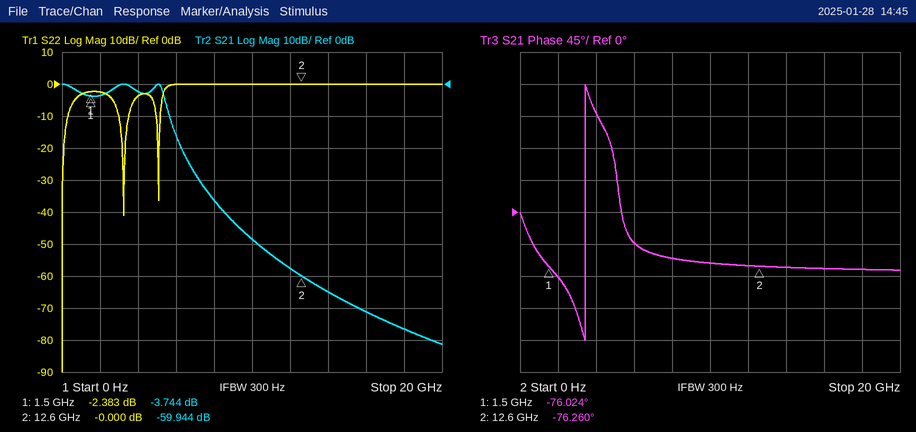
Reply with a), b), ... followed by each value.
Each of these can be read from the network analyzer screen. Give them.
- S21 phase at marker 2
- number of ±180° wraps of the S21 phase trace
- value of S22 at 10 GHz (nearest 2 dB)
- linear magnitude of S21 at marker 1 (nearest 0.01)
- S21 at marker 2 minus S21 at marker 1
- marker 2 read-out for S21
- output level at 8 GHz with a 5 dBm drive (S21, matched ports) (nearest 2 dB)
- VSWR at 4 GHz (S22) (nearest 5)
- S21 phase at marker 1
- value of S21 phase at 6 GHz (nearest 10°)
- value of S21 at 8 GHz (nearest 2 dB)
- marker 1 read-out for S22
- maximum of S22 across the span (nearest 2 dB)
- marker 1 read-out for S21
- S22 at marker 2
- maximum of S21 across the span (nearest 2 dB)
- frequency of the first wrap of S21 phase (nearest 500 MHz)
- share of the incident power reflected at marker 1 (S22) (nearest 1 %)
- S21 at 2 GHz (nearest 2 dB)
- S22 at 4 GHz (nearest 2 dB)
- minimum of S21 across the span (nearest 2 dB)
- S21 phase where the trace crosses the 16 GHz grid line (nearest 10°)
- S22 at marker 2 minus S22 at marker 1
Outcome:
a) -76.260°
b) 1
c) 0 dB
d) 0.65
e) -56.200 dB
f) -59.944 dB
g) -32 dBm
h) 5
i) -76.024°
j) -40°
k) -36 dB
l) -2.383 dB
m) 0 dB
n) -3.744 dB
o) -0.000 dB
p) 0 dB
q) 3.5 GHz
r) 58 %
s) -4 dB
t) -4 dB
u) -82 dB
v) -80°
w) 2.383 dB
